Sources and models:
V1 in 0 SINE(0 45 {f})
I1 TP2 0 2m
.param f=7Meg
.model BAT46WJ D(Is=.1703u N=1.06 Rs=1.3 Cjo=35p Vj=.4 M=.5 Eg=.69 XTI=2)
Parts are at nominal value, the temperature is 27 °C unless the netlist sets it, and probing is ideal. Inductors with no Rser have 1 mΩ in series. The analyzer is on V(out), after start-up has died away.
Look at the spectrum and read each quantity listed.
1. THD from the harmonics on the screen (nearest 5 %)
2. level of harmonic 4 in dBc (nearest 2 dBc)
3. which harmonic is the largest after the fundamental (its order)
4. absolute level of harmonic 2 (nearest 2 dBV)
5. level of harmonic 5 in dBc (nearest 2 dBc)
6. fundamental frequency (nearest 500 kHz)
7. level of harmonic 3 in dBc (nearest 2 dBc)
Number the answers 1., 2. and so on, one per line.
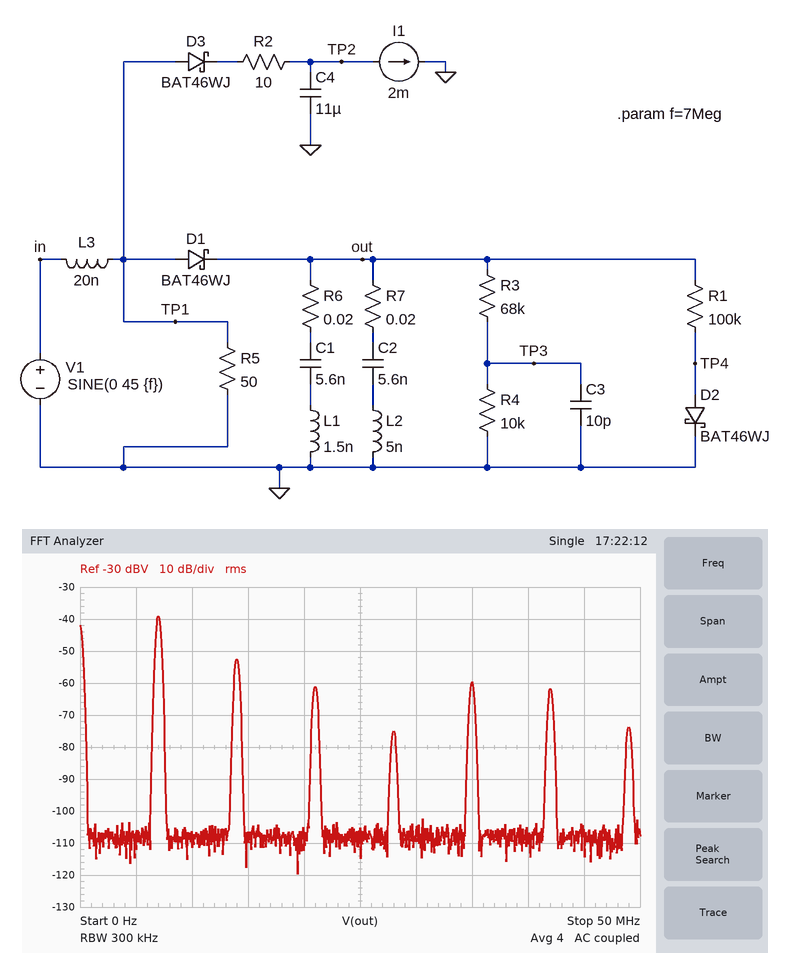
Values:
1. 25 %
2. -36 dBc
3. 2
4. -52 dBV
5. -20 dBc
6. 7.0 MHz
7. -22 dBc
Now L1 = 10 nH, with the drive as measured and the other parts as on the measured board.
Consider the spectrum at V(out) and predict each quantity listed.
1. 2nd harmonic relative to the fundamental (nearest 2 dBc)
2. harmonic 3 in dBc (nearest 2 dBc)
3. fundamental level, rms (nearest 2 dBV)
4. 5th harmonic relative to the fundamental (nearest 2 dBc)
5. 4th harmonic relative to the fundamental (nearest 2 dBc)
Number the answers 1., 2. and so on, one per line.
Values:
1. -16 dBc
2. -42 dBc
3. -40 dBV
4. -30 dBc
5. -32 dBc
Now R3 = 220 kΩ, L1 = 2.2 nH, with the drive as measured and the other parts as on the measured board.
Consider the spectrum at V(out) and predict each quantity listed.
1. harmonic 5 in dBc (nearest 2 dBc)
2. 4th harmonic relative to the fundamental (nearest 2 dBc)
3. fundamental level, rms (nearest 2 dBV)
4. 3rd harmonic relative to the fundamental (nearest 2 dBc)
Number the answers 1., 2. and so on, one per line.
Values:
1. -16 dBc
2. -38 dBc
3. -40 dBV
4. -24 dBc
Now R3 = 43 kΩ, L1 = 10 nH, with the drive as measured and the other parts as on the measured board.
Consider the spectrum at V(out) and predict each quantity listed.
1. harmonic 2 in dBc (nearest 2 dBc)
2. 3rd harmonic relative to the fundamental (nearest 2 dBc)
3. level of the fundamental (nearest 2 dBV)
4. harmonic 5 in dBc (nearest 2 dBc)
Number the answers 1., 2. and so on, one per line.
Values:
1. -14 dBc
2. -42 dBc
3. -40 dBV
4. -28 dBc
